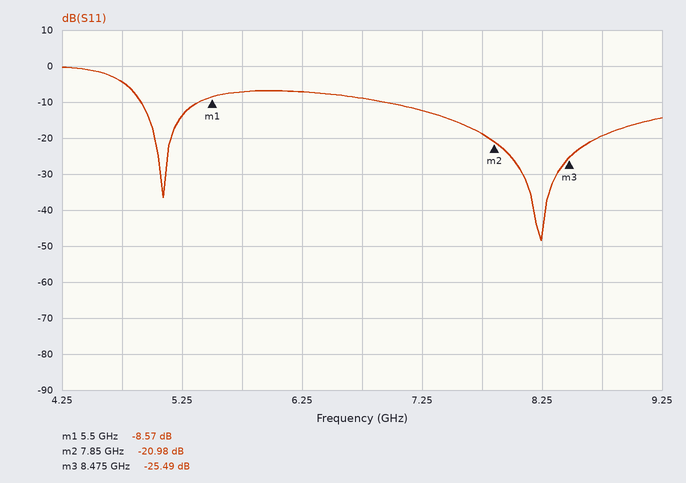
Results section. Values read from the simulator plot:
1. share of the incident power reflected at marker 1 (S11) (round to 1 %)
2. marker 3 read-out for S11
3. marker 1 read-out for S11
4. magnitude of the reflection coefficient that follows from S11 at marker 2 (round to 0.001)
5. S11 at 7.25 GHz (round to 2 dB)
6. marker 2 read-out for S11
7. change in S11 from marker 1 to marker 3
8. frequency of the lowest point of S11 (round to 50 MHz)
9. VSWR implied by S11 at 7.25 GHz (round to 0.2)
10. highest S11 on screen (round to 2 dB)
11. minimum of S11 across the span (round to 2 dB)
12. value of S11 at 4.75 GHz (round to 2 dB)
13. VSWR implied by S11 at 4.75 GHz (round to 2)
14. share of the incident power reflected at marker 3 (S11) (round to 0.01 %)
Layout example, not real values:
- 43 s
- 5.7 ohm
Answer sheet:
- 14 %
- -25.49 dB
- -8.57 dB
- 0.089
- -12 dB
- -20.98 dB
- -16.92 dB
- 8.25 GHz
- 1.6
- 0 dB
- -48 dB
- -4 dB
- 4
- 0.28 %
